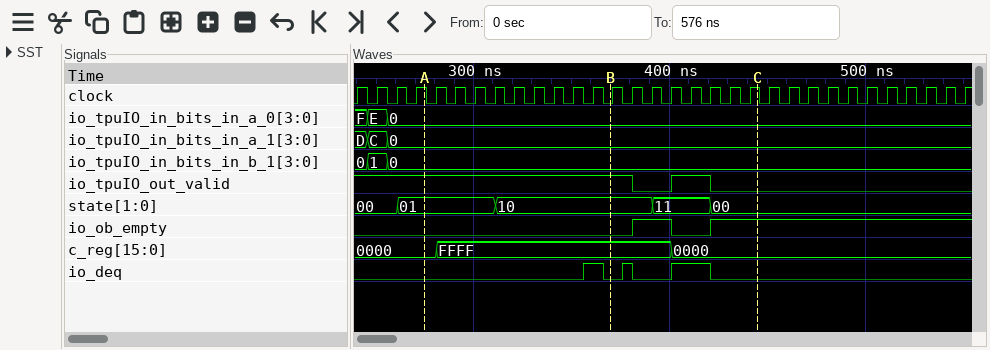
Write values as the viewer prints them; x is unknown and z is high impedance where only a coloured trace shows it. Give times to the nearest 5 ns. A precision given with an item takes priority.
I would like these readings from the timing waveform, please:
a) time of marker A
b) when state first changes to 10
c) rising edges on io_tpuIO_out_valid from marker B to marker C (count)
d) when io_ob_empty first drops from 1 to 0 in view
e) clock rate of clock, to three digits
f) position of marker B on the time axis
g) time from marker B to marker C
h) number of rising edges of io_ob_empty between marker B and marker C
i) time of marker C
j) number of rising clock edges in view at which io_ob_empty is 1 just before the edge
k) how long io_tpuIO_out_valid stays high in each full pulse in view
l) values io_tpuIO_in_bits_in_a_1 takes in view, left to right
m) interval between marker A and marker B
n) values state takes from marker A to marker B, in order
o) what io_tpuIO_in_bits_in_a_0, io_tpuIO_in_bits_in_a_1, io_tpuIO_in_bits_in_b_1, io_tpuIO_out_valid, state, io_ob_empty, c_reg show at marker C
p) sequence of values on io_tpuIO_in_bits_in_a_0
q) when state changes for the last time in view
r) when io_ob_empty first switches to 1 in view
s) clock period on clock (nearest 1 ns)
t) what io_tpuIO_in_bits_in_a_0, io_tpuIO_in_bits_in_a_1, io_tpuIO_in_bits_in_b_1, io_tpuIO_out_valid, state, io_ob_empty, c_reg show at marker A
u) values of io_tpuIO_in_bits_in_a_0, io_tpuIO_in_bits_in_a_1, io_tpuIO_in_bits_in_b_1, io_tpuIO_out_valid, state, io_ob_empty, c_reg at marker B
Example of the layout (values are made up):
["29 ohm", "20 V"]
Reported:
["275 ns", "310 ns", "1", "400 ns", "100 MHz", "370 ns", "75 ns", "2", "445 ns", "15", "20 ns", "D, C, 0", "95 ns", "01, 10", "io_tpuIO_in_bits_in_a_0=0, io_tpuIO_in_bits_in_a_1=0, io_tpuIO_in_bits_in_b_1=0, io_tpuIO_out_valid=0, state=00, io_ob_empty=1, c_reg=0000", "F, E, 0", "420 ns", "380 ns", "10 ns", "io_tpuIO_in_bits_in_a_0=0, io_tpuIO_in_bits_in_a_1=0, io_tpuIO_in_bits_in_b_1=0, io_tpuIO_out_valid=1, state=01, io_ob_empty=0, c_reg=0000", "io_tpuIO_in_bits_in_a_0=0, io_tpuIO_in_bits_in_a_1=0, io_tpuIO_in_bits_in_b_1=0, io_tpuIO_out_valid=1, state=10, io_ob_empty=0, c_reg=FFFF"]
